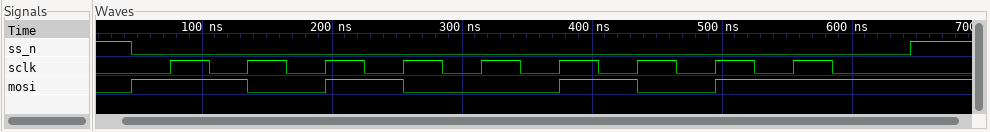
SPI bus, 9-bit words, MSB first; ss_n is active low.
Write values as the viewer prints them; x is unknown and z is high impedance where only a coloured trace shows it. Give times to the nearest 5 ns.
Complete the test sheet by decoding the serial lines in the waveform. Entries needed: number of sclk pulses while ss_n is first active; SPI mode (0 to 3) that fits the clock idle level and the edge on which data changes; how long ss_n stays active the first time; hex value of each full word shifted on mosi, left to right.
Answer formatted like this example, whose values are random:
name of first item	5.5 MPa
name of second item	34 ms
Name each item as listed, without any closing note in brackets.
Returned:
number of sclk pulses while ss_n is first active	9
SPI mode (0 to 3) that fits the clock idle level and the edge on which data changes	1
how long ss_n stays active the first time	600 ns
hex value of each full word shifted on mosi, left to right	14B
